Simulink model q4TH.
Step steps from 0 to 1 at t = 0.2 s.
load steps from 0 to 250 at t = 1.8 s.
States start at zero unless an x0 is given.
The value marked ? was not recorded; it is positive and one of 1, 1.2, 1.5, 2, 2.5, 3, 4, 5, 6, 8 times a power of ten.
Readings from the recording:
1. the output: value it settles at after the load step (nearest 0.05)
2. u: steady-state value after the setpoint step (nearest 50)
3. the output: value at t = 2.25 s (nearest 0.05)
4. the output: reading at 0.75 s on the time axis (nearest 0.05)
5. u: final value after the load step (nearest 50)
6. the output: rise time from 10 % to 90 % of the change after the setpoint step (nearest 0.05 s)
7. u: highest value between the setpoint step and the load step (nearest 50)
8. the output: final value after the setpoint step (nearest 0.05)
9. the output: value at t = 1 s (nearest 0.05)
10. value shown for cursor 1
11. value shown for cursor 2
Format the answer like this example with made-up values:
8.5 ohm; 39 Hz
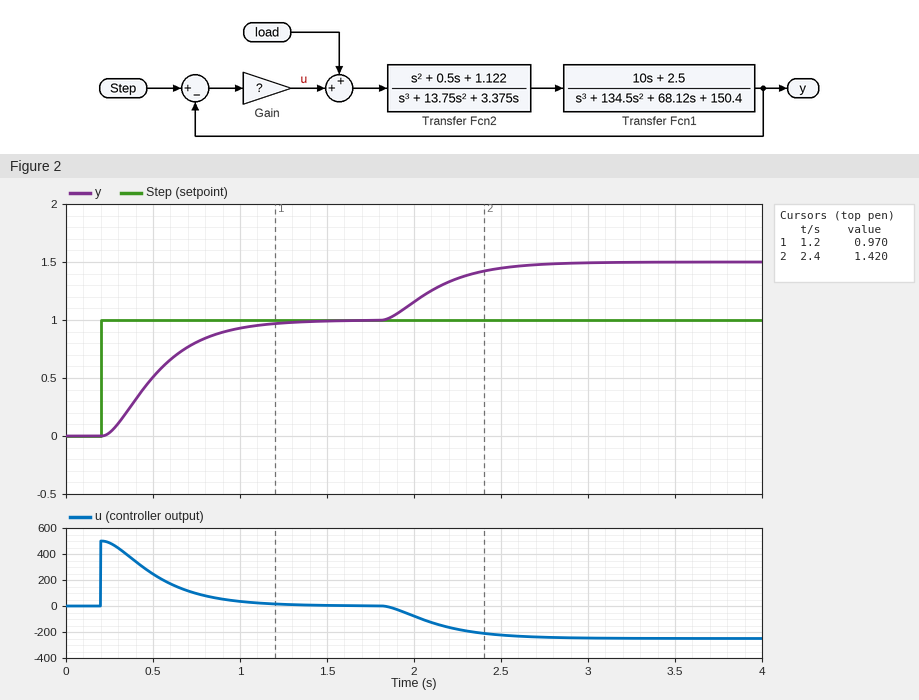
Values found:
1.50; 0; 1.35; 0.80; -250; 0.60 s; 500; 1.00; 0.95; 0.970; 1.420
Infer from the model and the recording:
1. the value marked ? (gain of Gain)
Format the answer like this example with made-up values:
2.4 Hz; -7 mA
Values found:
500
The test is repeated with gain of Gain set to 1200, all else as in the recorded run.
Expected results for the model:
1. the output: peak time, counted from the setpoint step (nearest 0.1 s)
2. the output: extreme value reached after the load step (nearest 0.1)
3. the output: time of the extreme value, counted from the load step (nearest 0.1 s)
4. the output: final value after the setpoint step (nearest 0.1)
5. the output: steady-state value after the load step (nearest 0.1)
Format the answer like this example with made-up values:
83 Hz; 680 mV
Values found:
0.5 s; 1.2; 0.5 s; 1.0; 1.2
